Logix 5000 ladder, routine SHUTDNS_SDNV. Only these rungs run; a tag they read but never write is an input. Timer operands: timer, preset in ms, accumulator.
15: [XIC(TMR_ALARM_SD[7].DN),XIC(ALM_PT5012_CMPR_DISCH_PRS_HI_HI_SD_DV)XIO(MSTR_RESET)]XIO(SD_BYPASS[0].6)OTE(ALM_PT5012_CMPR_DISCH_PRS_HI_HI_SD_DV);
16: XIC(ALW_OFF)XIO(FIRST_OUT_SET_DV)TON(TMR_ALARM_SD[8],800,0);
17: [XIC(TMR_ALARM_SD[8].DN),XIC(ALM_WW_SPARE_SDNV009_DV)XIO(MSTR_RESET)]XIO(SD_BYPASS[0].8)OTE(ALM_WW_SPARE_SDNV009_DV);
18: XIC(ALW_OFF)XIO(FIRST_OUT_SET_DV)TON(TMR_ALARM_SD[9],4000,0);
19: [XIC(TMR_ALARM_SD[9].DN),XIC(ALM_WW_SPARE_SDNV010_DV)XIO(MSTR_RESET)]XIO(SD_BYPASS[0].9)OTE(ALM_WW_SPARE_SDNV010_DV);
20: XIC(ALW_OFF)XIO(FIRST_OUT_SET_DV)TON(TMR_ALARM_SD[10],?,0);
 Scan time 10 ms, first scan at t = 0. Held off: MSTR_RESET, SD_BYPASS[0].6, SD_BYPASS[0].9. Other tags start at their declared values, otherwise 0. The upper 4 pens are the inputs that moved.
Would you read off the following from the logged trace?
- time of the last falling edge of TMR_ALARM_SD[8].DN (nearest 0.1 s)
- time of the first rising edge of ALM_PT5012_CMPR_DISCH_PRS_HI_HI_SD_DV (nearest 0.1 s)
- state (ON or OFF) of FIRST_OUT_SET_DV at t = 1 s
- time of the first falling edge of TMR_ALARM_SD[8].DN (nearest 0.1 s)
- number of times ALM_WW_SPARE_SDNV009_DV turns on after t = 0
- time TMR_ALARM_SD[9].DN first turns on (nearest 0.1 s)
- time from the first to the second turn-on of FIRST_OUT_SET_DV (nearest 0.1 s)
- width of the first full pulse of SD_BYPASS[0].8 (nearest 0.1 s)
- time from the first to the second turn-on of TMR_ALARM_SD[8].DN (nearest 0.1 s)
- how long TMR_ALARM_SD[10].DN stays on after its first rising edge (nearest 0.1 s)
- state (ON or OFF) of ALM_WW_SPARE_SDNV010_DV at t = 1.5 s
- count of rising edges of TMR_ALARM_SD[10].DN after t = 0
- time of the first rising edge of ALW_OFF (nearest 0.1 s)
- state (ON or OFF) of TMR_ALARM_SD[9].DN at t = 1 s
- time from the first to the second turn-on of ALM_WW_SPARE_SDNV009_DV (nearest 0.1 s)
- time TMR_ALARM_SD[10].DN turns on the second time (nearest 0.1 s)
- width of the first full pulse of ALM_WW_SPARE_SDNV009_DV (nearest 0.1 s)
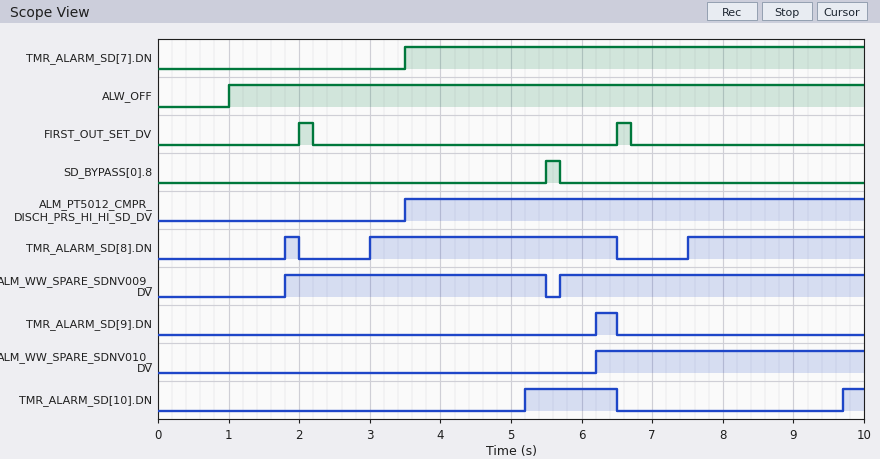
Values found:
6.5 s
3.5 s
OFF
2.0 s
2
6.2 s
4.5 s
0.2 s
1.2 s
1.3 s
OFF
2
1.0 s
OFF
3.9 s
9.7 s
3.7 s
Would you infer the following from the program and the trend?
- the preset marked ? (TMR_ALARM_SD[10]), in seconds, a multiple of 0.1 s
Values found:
3.0 s
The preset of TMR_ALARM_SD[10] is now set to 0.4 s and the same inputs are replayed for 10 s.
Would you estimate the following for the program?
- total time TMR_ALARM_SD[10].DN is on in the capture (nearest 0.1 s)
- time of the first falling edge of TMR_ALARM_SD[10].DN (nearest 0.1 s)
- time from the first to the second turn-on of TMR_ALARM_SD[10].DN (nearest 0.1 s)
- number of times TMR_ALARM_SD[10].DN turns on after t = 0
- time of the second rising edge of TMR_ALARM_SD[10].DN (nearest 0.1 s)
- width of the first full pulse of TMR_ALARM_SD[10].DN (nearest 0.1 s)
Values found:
7.4 s
2.0 s
1.2 s
3
2.6 s
0.6 s
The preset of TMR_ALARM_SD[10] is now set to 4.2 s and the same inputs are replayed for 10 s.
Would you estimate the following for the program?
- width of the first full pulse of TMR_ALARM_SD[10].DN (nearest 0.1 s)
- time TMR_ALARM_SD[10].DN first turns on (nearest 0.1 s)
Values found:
0.1 s
6.4 s
